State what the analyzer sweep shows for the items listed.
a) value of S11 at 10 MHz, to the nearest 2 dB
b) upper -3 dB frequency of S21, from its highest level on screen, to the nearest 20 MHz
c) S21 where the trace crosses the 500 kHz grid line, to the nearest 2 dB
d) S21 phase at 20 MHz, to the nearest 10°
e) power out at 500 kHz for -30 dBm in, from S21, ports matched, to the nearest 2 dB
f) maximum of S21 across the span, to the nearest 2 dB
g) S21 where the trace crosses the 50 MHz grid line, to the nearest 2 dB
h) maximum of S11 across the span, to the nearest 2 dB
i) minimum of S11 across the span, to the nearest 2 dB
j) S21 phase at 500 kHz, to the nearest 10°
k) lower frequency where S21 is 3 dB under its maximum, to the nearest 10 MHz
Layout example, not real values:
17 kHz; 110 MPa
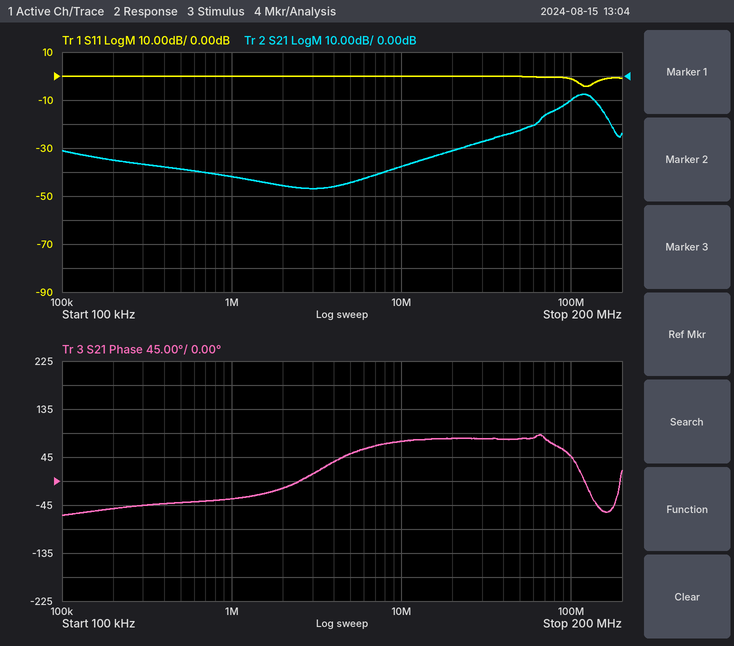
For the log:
0 dB; 140 MHz; -38 dB; 80°; -68 dBm; -8 dB; -22 dB; 0 dB; -4 dB; -40°; 100 MHz
